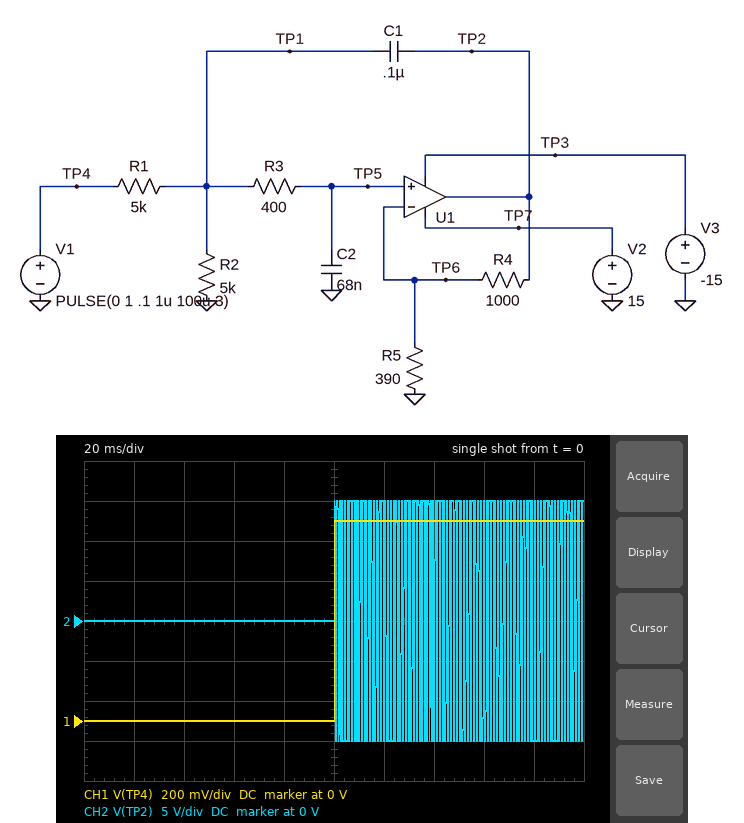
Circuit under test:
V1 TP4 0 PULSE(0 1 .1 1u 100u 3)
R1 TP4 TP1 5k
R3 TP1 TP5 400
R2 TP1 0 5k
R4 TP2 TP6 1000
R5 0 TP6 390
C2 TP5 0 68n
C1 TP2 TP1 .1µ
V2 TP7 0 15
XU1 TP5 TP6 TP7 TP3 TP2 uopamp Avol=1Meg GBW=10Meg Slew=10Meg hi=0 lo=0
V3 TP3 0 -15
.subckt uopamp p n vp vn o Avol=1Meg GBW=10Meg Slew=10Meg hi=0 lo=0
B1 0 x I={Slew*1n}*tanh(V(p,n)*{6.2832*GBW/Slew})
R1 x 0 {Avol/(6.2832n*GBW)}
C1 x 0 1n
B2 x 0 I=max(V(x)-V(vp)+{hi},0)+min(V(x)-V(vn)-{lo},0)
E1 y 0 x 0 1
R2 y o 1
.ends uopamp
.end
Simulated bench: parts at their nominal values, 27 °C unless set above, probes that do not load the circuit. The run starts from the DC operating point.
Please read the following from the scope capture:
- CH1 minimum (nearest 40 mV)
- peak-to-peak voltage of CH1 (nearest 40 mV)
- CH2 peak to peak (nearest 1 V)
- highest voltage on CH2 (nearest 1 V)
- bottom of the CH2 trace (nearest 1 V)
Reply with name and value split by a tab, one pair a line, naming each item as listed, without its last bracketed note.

CH1 minimum	0 V
peak-to-peak voltage of CH1	1.00 V
CH2 peak to peak	30 V
highest voltage on CH2	15 V
bottom of the CH2 trace	-15 V
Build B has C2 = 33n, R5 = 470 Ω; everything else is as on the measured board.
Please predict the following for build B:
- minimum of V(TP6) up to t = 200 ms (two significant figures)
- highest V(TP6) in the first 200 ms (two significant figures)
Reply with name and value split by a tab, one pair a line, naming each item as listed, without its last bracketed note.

minimum of V(TP6) up to t = 200 ms	-4.8 V
highest V(TP6) in the first 200 ms	4.8 V
